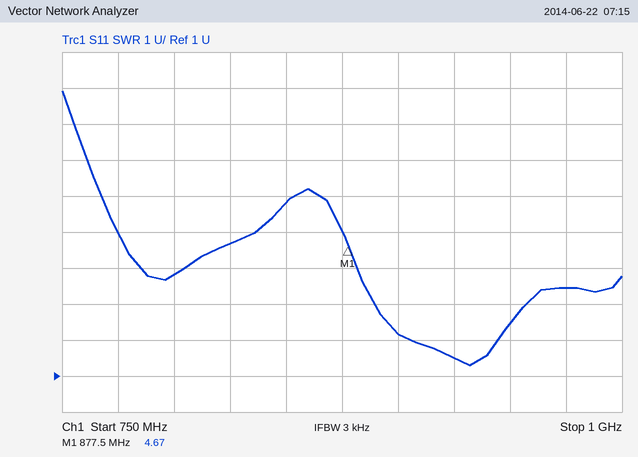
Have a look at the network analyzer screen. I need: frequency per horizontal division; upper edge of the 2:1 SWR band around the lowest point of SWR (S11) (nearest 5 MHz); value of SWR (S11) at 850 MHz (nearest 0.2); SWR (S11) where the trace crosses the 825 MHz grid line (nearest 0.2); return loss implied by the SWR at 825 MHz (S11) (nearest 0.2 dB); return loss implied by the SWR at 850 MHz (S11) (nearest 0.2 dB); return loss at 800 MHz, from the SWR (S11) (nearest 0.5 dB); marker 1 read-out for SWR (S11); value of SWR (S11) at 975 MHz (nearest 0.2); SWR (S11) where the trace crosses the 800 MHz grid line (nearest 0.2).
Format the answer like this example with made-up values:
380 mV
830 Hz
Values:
25 MHz
945 MHz
5.8
4.6
3.8 dB
3.0 dB
4.5 dB
4.67
3.4
3.8
